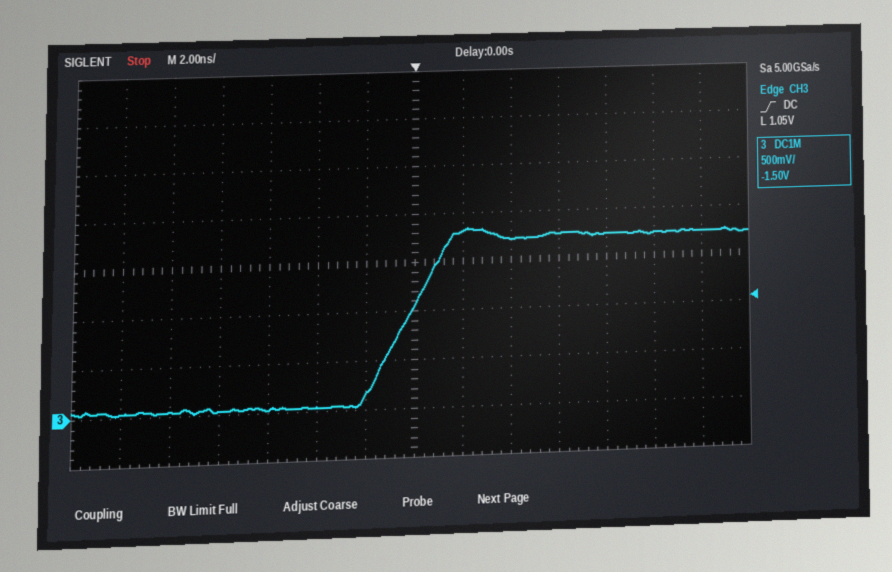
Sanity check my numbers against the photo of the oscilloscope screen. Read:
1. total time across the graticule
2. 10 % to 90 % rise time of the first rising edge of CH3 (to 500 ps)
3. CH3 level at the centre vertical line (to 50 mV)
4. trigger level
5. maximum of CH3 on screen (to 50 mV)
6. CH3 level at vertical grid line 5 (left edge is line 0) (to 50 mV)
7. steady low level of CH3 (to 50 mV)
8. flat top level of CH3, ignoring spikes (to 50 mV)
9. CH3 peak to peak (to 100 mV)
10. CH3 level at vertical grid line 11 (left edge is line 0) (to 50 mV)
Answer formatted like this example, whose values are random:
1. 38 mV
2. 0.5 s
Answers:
1. 28 ns
2. 3.0 ns
3. 1.05 V
4. 1.05 V
5. 1.85 V
6. 50 mV
7. 50 mV
8. 1.75 V
9. 1.80 V
10. 1.75 V
